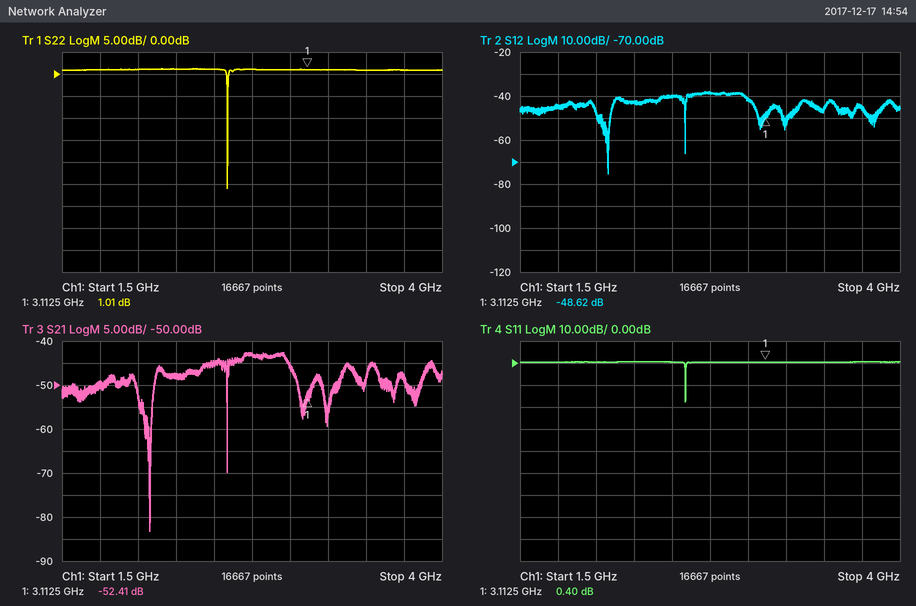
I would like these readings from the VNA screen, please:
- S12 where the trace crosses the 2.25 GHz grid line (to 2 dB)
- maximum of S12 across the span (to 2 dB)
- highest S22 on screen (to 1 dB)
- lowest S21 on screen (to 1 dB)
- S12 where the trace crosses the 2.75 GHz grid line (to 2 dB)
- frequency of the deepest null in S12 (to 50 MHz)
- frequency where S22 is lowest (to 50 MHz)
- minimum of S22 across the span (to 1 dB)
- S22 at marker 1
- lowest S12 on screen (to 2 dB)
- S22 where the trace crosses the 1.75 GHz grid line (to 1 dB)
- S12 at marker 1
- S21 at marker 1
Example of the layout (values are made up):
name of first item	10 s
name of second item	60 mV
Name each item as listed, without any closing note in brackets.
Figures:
S12 where the trace crosses the 2.25 GHz grid line	-42 dB
maximum of S12 across the span	-38 dB
highest S22 on screen	1 dB
lowest S21 on screen	-83 dB
S12 where the trace crosses the 2.75 GHz grid line	-38 dB
frequency of the deepest null in S12	2.10 GHz
frequency where S22 is lowest	2.60 GHz
minimum of S22 across the span	-26 dB
S22 at marker 1	1.01 dB
lowest S12 on screen	-76 dB
S22 where the trace crosses the 1.75 GHz grid line	1 dB
S12 at marker 1	-48.62 dB
S21 at marker 1	-52.41 dB
